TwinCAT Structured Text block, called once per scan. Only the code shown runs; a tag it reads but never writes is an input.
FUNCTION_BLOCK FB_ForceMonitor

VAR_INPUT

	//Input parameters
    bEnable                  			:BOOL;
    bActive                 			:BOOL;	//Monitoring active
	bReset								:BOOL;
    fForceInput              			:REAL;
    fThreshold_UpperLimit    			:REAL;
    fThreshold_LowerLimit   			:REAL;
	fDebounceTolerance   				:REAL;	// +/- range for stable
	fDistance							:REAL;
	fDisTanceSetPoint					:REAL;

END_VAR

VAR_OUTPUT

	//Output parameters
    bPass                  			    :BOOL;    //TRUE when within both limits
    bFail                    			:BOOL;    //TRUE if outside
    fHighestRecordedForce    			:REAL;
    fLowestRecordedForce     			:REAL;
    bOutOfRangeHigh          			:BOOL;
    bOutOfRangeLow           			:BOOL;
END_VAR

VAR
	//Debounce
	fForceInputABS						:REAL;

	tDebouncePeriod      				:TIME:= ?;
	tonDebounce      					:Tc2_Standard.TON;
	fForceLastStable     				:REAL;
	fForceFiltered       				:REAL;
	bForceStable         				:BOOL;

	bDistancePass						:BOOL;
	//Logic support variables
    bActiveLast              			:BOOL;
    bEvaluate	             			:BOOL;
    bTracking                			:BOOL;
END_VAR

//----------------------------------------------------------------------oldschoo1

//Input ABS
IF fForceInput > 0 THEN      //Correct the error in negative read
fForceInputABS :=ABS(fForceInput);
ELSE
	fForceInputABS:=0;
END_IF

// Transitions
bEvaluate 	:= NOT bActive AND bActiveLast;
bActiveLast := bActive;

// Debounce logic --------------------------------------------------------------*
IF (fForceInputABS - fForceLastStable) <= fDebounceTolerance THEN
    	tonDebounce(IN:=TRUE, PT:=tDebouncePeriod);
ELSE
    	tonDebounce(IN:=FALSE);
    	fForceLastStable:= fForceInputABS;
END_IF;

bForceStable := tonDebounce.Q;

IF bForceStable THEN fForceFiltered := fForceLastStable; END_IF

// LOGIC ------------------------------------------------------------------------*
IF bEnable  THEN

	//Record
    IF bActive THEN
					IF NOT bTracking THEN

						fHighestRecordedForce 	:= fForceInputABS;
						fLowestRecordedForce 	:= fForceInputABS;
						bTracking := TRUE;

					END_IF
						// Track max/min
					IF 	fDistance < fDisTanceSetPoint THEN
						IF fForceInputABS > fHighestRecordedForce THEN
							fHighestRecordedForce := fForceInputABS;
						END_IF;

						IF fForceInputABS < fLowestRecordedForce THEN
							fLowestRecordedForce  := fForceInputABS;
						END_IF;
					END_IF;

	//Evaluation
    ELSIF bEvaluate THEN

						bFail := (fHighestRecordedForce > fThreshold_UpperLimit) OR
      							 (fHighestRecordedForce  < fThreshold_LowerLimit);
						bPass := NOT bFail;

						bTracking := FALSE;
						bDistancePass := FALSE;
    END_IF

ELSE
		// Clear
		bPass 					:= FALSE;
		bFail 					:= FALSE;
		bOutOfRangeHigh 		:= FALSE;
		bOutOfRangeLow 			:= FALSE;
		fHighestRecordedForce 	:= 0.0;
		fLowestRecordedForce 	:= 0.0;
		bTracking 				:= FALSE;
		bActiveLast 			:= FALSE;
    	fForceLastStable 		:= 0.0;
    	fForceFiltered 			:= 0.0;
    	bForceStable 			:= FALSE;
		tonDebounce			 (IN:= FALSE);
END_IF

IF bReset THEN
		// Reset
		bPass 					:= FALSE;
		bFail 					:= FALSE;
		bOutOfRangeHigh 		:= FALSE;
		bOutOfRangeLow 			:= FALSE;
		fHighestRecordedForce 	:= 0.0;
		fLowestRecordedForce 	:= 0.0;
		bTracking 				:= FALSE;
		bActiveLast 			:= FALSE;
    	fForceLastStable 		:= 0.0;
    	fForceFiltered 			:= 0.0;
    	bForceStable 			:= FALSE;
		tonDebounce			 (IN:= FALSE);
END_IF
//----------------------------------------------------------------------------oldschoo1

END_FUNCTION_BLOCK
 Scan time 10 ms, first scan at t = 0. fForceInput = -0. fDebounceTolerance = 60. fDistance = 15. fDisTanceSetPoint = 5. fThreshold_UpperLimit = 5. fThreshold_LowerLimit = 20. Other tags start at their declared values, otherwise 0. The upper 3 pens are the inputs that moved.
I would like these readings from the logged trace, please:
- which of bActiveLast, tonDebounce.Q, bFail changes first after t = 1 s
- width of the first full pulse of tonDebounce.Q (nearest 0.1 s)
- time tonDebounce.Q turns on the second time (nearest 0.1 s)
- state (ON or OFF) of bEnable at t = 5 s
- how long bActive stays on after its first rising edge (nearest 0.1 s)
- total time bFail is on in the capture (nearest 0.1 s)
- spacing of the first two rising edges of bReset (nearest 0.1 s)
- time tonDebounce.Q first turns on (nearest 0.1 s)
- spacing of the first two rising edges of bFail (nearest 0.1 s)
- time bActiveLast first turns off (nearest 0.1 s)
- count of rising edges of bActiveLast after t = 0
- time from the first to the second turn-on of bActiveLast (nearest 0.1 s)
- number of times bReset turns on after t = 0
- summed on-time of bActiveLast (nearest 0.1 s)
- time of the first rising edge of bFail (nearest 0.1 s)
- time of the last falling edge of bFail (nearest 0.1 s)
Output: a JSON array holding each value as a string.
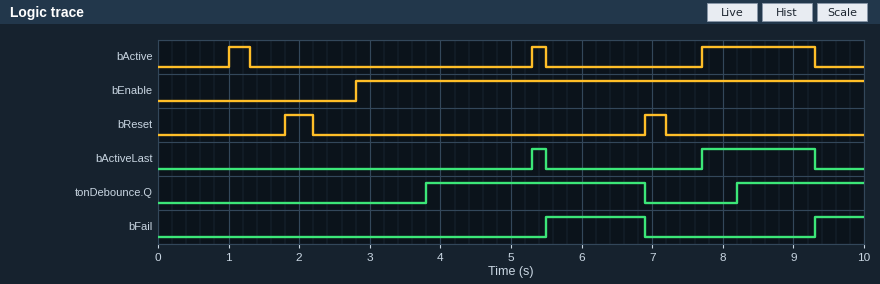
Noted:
["tonDebounce.Q", "3.1 s", "8.2 s", "ON", "0.3 s", "2.1 s", "5.1 s", "3.8 s", "3.8 s", "5.5 s", "2", "2.4 s", "2", "1.8 s", "5.5 s", "6.9 s"]
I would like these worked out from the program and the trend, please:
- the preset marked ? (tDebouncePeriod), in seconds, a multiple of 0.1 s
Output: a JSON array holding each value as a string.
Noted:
["1.0 s"]
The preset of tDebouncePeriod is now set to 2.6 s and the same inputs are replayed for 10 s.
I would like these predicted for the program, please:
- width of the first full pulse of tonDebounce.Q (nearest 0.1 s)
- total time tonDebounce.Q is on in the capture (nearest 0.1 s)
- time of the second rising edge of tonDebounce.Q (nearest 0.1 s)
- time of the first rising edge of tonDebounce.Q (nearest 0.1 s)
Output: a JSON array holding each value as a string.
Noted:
["1.5 s", "1.7 s", "9.8 s", "5.4 s"]
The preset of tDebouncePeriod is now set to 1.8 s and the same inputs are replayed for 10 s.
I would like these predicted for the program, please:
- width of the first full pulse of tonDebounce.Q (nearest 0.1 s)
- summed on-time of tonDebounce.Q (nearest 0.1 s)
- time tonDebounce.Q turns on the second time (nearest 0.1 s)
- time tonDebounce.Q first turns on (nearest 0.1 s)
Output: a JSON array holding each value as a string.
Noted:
["2.3 s", "3.3 s", "9.0 s", "4.6 s"]
